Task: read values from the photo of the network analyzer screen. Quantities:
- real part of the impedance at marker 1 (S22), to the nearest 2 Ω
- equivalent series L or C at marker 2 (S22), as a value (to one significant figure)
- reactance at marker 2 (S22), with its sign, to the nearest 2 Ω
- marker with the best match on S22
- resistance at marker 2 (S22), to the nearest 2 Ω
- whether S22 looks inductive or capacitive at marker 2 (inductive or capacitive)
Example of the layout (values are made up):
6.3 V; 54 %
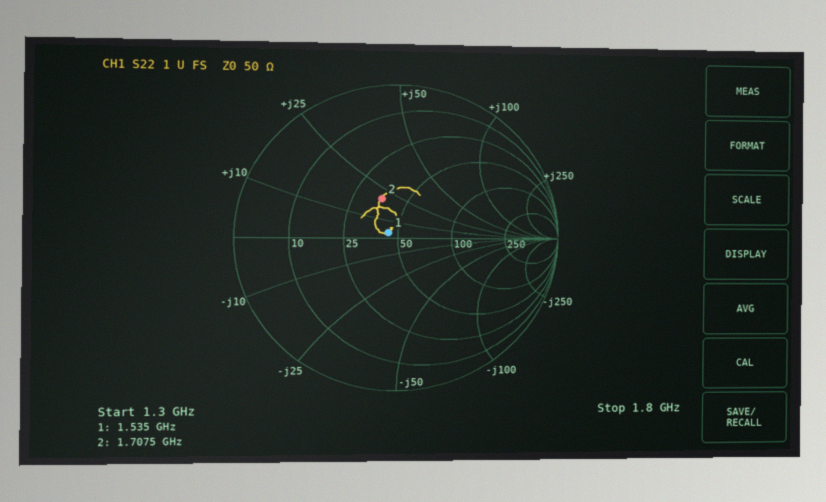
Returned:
44 Ω; 2 nH; +20 Ω; marker 1; 36 Ω; inductive
